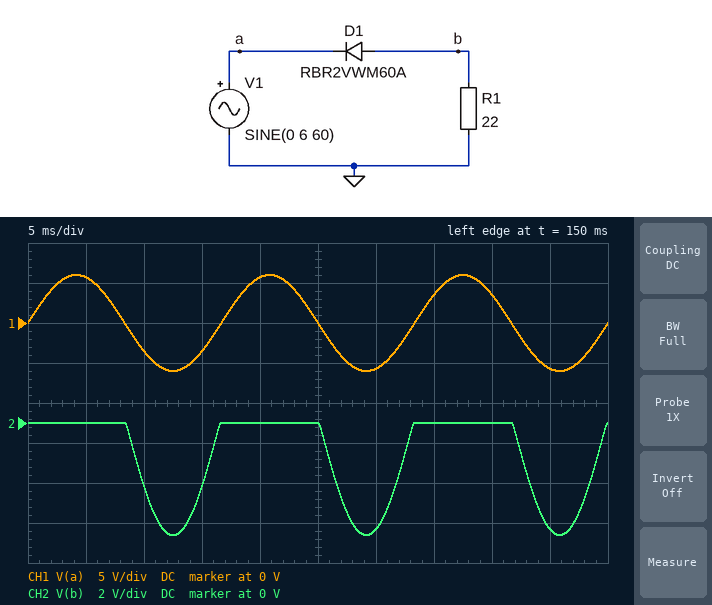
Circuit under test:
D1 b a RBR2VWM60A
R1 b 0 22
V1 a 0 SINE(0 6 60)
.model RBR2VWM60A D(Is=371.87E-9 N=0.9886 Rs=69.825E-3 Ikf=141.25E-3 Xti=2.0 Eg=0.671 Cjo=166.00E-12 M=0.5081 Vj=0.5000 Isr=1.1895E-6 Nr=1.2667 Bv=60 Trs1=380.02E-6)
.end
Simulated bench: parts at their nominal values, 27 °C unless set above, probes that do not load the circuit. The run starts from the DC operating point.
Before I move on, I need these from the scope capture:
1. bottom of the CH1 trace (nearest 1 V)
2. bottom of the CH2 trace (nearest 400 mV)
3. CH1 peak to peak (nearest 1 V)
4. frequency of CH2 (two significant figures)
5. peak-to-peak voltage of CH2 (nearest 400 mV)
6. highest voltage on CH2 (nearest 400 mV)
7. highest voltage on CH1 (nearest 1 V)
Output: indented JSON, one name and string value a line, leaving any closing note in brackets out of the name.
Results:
{
  "bottom of the CH1 trace": "-6 V",
  "bottom of the CH2 trace": "-5.6 V",
  "CH1 peak to peak": "12 V",
  "frequency of CH2": "60 Hz",
  "peak-to-peak voltage of CH2": "5.6 V",
  "highest voltage on CH2": "0 V",
  "highest voltage on CH1": "6 V"
}
